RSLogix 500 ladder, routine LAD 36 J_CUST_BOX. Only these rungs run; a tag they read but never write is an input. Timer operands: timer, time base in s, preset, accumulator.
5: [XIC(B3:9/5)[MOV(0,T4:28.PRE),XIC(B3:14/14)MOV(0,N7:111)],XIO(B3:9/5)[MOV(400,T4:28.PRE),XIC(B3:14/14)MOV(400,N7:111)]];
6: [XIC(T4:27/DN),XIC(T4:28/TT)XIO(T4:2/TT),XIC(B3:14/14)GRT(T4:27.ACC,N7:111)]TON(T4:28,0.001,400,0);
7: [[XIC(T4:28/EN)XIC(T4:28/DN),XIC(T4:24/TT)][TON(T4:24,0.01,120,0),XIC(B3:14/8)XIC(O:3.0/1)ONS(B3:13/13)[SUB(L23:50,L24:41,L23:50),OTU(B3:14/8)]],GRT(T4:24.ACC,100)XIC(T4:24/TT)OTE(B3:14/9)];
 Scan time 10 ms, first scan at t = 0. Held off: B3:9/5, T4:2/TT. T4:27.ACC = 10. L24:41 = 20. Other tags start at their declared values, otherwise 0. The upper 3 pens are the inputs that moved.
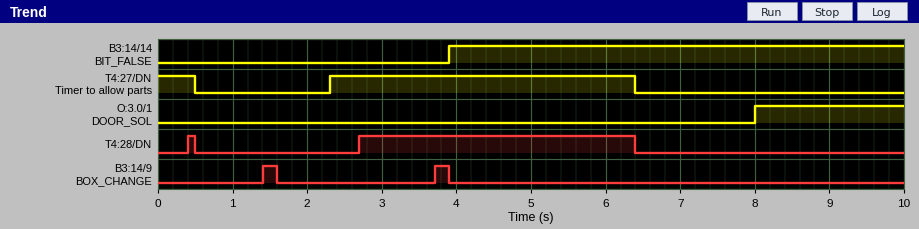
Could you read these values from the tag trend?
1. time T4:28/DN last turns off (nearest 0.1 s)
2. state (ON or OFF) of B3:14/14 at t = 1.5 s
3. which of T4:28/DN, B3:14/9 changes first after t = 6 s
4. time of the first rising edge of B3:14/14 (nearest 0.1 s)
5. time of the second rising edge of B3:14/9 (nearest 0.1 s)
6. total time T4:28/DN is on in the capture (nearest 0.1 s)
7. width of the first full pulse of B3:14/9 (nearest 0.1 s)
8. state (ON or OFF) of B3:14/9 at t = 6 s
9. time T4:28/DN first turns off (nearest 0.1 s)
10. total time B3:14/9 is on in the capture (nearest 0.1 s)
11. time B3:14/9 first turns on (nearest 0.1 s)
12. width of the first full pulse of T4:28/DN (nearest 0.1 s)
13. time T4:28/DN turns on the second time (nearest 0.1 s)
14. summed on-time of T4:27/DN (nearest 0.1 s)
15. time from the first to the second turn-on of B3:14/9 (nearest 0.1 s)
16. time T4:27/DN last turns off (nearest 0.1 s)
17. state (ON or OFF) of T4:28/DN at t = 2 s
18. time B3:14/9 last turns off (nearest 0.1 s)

6.4 s
OFF
T4:28/DN
3.9 s
3.7 s
3.8 s
0.2 s
OFF
0.5 s
0.4 s
1.4 s
0.1 s
2.7 s
4.6 s
2.3 s
6.4 s
OFF
3.9 s
